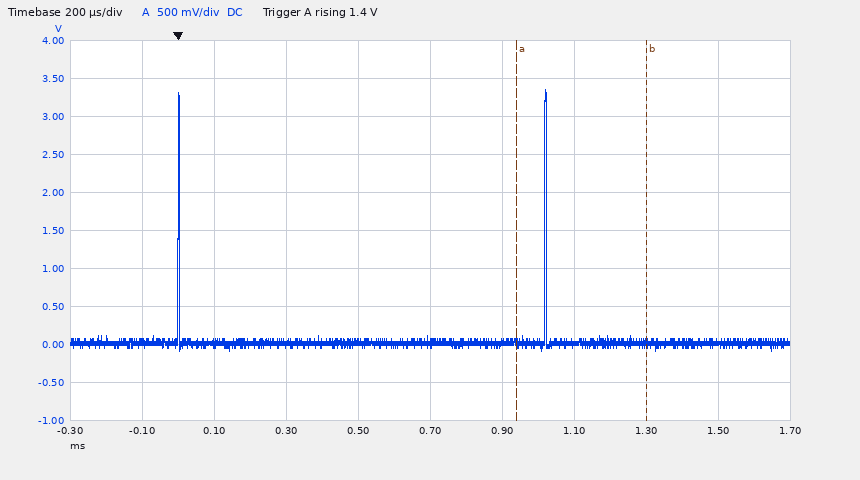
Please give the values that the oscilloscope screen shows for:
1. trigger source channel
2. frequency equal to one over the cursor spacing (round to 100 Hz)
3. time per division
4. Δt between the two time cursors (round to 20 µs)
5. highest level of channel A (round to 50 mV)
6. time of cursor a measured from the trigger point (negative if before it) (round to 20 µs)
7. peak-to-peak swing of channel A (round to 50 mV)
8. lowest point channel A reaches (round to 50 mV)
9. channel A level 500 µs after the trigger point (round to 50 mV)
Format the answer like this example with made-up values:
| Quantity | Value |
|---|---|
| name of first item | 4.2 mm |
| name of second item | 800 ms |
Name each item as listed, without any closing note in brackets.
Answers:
| Quantity | Value |
|---|---|
| trigger source channel | channel A |
| frequency equal to one over the cursor spacing | 2.8 kHz |
| time per division | 200 µs |
| Δt between the two time cursors | 360 µs |
| highest level of channel A | 3.35 V |
| time of cursor a measured from the trigger point (negative if before it) | +940 µs |
| peak-to-peak swing of channel A | 3.45 V |
| lowest point channel A reaches | -100 mV |
| channel A level 500 µs after the trigger point | 50 mV |
